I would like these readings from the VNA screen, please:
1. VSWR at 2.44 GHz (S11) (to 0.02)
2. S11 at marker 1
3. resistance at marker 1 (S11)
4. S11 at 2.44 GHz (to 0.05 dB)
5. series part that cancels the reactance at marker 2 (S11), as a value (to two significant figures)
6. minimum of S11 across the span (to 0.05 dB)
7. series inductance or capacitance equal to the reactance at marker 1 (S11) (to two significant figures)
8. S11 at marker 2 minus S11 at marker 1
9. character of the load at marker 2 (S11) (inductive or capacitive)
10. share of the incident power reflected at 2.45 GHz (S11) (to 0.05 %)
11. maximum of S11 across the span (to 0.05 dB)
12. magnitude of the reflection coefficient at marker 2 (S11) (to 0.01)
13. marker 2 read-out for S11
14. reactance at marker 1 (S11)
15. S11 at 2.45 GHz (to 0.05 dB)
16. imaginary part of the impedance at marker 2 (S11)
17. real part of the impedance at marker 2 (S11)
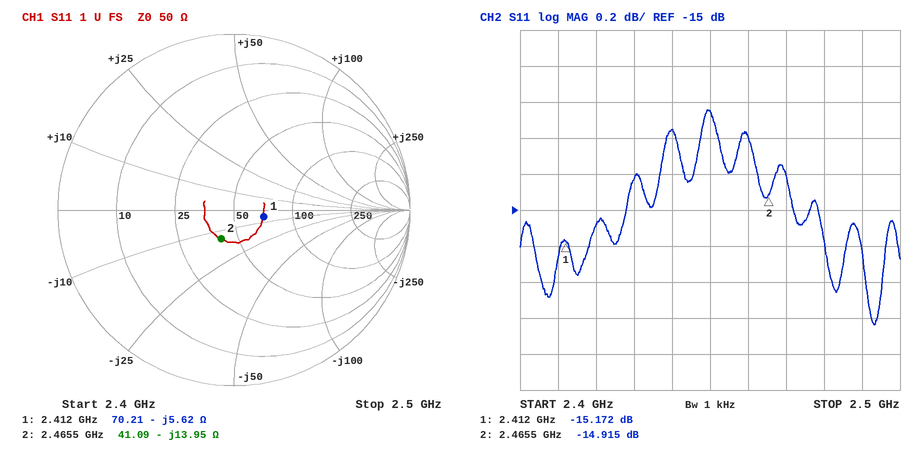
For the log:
1.46
-15.172 dB
70.21 Ω
-14.55 dB
900 pH
-15.65 dB
12 pF
0.257 dB
capacitive
3.60 %
-14.45 dB
0.18
-14.915 dB
-5.62 Ω
-14.45 dB
-13.95 Ω
41.09 Ω
